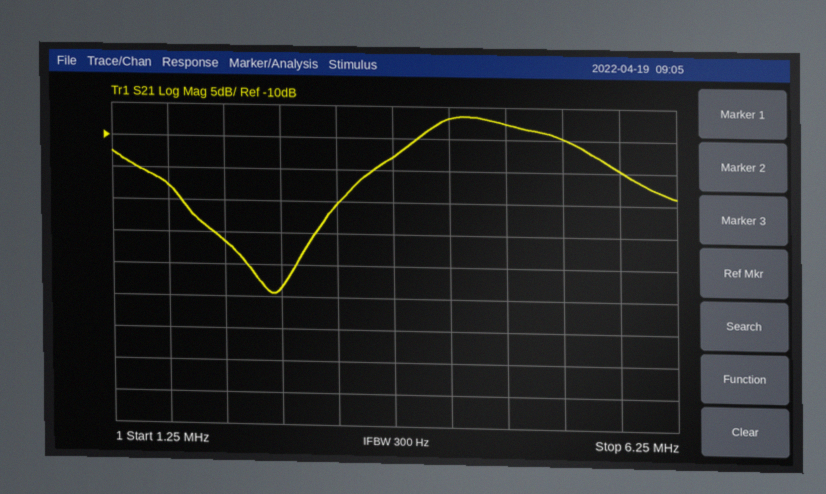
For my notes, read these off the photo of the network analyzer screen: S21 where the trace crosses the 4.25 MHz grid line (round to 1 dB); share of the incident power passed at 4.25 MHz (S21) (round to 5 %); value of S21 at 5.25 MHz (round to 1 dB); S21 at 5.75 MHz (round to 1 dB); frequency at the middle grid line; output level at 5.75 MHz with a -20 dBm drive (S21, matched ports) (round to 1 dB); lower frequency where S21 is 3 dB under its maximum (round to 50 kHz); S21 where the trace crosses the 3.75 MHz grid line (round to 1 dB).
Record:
-7 dB
20 %
-10 dB
-15 dB
3.75 MHz
-35 dBm
4.00 MHz
-13 dB
